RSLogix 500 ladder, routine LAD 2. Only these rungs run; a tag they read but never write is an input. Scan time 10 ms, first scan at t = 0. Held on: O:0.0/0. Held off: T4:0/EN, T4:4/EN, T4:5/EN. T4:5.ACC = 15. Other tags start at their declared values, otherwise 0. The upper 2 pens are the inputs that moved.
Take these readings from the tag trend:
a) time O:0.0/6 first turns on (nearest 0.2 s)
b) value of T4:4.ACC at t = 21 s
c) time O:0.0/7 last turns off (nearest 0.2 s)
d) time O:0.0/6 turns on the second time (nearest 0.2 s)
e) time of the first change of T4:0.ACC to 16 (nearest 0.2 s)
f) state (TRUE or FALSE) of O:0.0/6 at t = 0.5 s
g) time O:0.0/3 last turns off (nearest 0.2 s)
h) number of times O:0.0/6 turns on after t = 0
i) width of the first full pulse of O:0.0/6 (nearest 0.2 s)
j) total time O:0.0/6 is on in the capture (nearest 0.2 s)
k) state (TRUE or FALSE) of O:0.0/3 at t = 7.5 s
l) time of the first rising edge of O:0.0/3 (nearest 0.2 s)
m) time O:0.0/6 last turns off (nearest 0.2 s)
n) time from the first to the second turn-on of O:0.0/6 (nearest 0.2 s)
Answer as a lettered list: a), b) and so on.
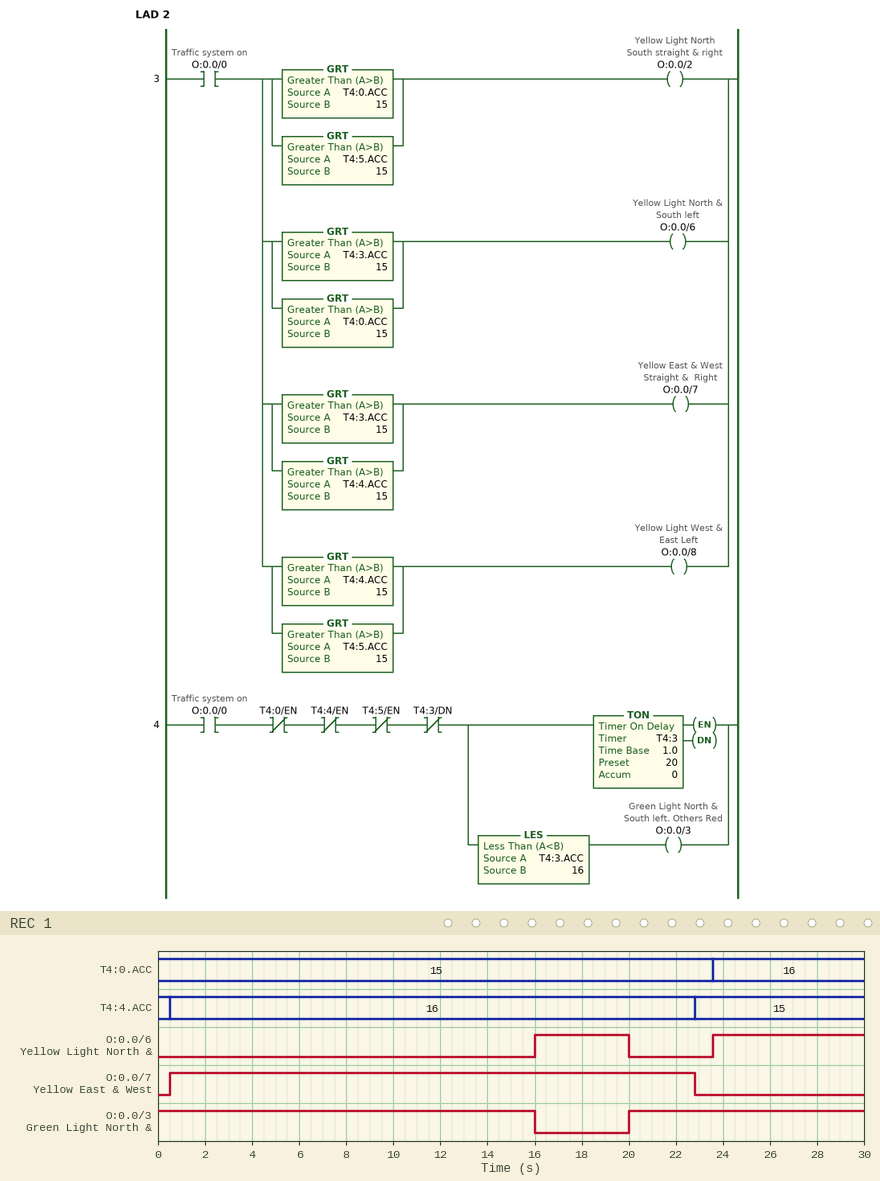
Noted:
a) 16.0 s
b) 16
c) 22.8 s
d) 23.6 s
e) 23.6 s
f) FALSE
g) 16.0 s
h) 2
i) 4.0 s
j) 10.4 s
k) TRUE
l) 20.0 s
m) 20.0 s
n) 7.6 s
